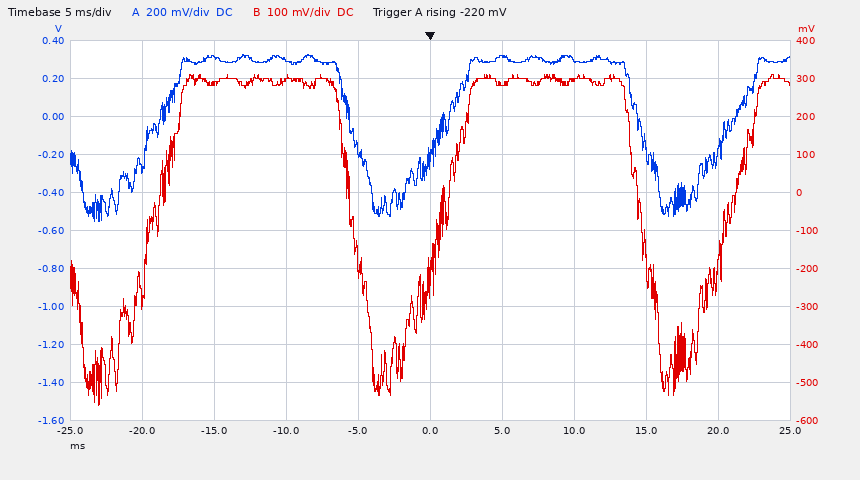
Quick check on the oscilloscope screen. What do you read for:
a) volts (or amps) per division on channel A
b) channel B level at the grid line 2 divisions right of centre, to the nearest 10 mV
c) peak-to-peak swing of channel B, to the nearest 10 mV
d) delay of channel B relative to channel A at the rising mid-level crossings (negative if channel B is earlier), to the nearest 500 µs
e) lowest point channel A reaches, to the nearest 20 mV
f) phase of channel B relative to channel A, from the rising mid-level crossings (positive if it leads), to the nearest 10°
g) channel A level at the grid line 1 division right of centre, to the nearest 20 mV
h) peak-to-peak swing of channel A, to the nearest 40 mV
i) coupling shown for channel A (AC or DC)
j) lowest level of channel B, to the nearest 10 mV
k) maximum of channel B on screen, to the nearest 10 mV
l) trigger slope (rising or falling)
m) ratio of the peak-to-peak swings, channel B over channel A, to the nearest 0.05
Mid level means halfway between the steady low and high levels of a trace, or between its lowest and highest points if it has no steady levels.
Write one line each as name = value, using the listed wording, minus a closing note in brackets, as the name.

volts (or amps) per division on channel A = 200 mV
channel B level at the grid line 2 divisions right of centre, to the nearest 10 mV = 300 mV
peak-to-peak swing of channel B, to the nearest 10 mV = 870 mV
delay of channel B relative to channel A at the rising mid-level crossings (negative if channel B is earlier), to the nearest 500 µs = 0.0 ms
lowest point channel A reaches, to the nearest 20 mV = -560 mV
phase of channel B relative to channel A, from the rising mid-level crossings (positive if it leads), to the nearest 10° = 0°
channel A level at the grid line 1 division right of centre, to the nearest 20 mV = 320 mV
peak-to-peak swing of channel A, to the nearest 40 mV = 880 mV
coupling shown for channel A = DC
lowest level of channel B, to the nearest 10 mV = -560 mV
maximum of channel B on screen, to the nearest 10 mV = 310 mV
trigger slope = rising
ratio of the peak-to-peak swings, channel B over channel A, to the nearest 0.05 = 1.00
